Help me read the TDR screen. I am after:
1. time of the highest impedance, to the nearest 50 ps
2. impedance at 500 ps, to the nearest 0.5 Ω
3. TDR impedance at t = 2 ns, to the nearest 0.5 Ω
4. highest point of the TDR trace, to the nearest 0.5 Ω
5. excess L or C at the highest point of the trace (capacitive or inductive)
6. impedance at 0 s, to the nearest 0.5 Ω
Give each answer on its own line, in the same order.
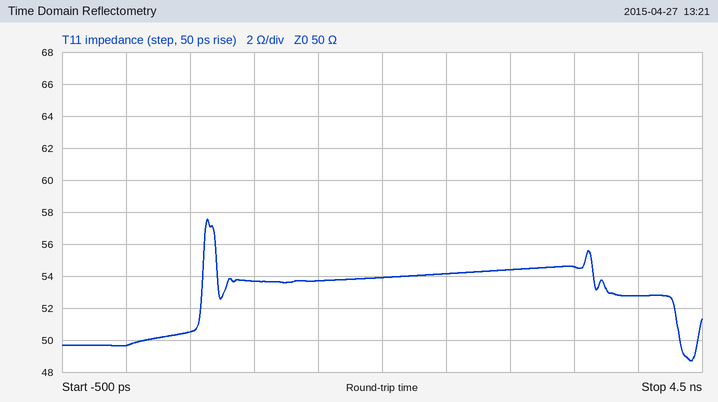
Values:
650 ps
50.5 Ω
54.0 Ω
57.5 Ω
inductive
49.5 Ω
